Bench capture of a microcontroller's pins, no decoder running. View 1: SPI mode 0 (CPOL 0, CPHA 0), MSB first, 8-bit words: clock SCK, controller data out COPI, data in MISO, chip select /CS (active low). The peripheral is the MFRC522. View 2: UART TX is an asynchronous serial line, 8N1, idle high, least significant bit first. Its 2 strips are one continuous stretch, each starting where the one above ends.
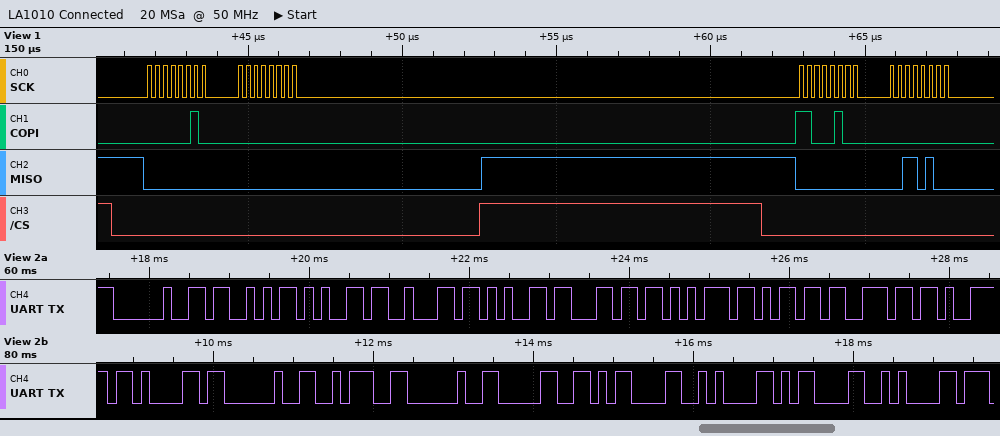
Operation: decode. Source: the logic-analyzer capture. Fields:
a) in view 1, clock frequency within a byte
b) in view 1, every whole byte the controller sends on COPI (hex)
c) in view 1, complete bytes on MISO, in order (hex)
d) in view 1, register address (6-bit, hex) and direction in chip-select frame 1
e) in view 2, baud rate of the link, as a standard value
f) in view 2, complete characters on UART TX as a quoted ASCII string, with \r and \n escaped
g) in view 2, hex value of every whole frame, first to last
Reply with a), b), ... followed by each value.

a) 4 MHz
b) 02 00 C4 00
c) 00 00 00 34
d) 0x01 write
e) 9600 baud
f) " Sebelumnya : 0\r\n\r\n"
g) 20 53 65 62 65 6C 75 6D 6E 79 61 20 3A 20 30 0D 0A 0D 0A
